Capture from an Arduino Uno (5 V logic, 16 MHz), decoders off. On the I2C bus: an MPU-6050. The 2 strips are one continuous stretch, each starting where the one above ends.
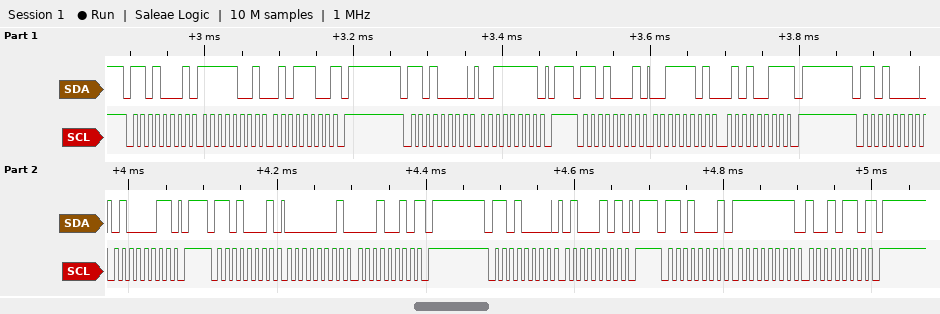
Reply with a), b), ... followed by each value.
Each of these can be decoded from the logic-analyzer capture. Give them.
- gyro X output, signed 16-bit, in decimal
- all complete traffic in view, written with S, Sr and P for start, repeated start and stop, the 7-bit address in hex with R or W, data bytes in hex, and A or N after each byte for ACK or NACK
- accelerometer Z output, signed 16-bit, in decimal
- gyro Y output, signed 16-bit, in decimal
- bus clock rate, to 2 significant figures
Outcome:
a) 274
b) S 68R A F9 A 5C N P S 68W A 3F A P S 68R A 3D A 53 N P S 68W A 43 A P S 68R A 01 A 12 N P S 68W A 45 A P S 68R A FF A 96 N P
c) 15699
d) -106
e) 100 kHz
